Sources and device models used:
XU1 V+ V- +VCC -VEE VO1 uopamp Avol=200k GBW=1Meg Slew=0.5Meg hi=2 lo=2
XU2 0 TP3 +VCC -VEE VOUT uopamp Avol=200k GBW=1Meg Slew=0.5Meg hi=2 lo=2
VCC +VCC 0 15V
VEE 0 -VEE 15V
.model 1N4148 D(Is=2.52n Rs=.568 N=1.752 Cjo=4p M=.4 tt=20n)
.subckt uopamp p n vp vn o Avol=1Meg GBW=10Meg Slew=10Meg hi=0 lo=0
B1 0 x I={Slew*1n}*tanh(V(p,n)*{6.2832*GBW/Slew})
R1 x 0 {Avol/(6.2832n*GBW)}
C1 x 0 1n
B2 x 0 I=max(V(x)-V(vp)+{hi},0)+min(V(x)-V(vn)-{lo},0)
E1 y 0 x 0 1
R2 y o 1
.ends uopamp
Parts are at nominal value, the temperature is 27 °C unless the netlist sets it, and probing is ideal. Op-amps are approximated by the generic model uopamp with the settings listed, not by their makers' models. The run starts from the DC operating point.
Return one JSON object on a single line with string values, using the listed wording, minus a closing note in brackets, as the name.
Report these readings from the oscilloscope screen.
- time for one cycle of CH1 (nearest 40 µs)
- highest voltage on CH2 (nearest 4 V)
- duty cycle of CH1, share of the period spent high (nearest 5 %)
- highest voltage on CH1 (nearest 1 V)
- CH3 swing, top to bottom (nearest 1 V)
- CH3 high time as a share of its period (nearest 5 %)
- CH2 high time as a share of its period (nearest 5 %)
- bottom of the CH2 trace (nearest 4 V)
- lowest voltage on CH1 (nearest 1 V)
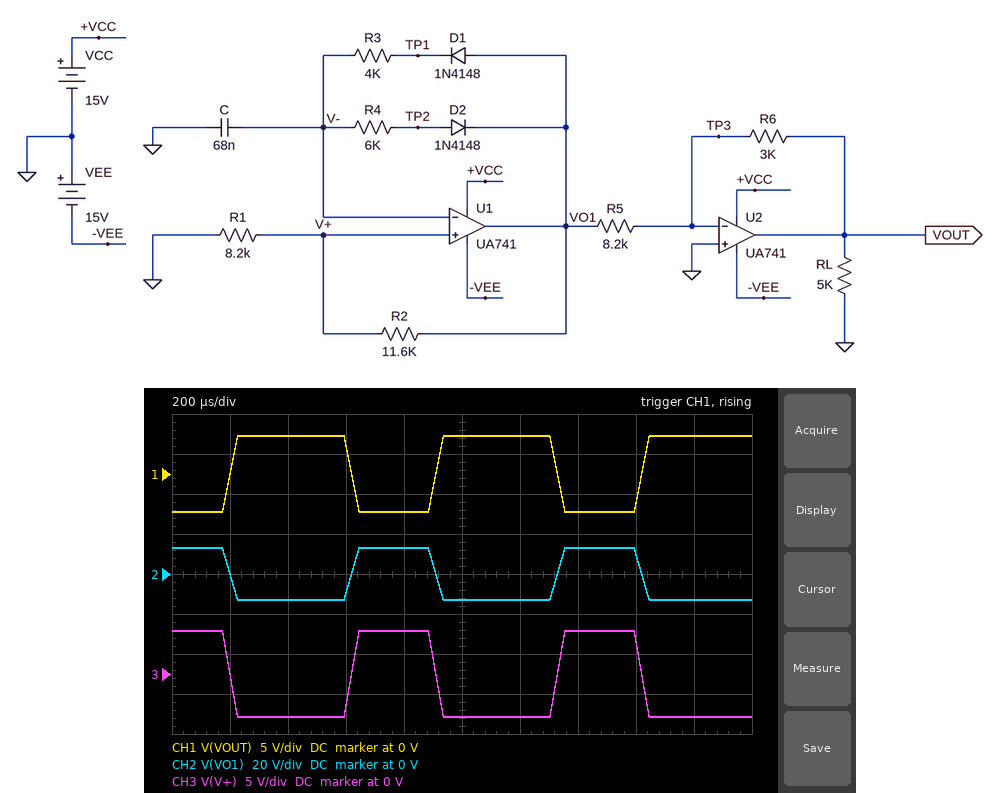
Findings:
{"time for one cycle of CH1": "720 µs", "highest voltage on CH2": "12 V", "duty cycle of CH1, share of the period spent high": "60 %", "highest voltage on CH1": "5 V", "CH3 swing, top to bottom": "11 V", "CH3 high time as a share of its period": "40 %", "CH2 high time as a share of its period": "40 %", "bottom of the CH2 trace": "-12 V", "lowest voltage on CH1": "-5 V"}
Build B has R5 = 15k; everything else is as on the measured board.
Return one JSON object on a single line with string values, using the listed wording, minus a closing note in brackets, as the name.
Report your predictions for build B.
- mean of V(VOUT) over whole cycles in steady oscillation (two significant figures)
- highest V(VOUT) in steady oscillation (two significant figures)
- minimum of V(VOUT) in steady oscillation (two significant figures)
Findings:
{"mean of V(VOUT) over whole cycles in steady oscillation": "470 mV", "highest V(VOUT) in steady oscillation": "2.6 V", "minimum of V(VOUT) in steady oscillation": "-2.6 V"}
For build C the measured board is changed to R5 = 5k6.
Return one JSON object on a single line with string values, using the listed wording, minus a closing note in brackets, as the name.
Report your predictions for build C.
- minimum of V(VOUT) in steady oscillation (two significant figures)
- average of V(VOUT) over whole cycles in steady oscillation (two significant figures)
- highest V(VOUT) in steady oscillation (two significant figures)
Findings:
{"minimum of V(VOUT) in steady oscillation": "-7.0 V", "average of V(VOUT) over whole cycles in steady oscillation": "1.3 V", "highest V(VOUT) in steady oscillation": "7.0 V"}
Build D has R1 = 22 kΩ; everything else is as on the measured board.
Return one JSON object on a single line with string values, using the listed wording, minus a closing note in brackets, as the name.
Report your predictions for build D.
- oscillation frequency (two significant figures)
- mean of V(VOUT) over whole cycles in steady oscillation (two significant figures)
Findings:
{"oscillation frequency": "830 Hz", "mean of V(VOUT) over whole cycles in steady oscillation": "900 mV"}
